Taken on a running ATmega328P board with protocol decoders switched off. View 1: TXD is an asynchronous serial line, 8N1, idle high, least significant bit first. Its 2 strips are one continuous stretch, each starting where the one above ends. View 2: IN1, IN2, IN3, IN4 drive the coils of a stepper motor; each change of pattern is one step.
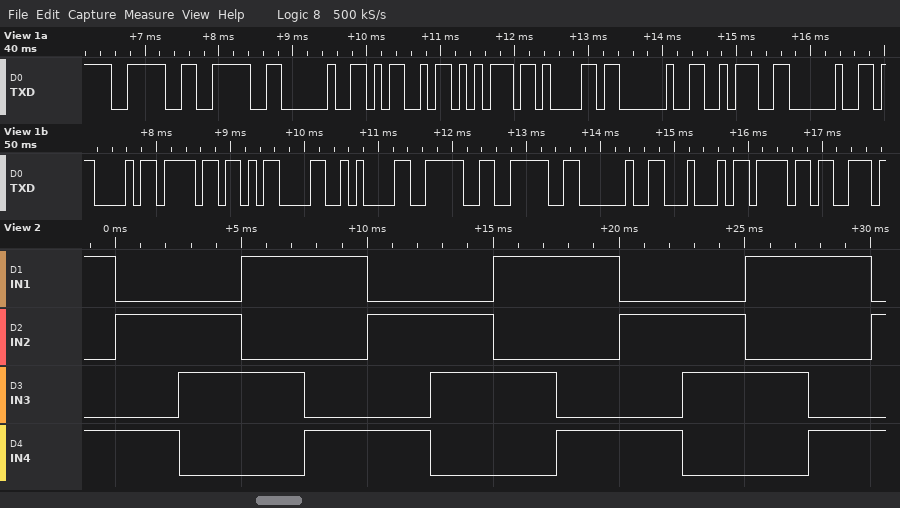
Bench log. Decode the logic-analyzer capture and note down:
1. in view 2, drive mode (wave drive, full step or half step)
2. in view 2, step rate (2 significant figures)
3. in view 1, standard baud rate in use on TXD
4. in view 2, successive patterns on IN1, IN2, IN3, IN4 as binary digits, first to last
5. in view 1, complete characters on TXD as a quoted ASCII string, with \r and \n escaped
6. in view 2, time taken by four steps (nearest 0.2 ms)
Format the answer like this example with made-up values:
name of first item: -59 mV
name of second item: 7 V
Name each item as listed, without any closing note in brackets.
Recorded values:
in view 2, drive mode: full step
in view 2, step rate: 400 steps/s
in view 1, standard baud rate in use on TXD: 9600 baud
in view 2, successive patterns on IN1, IN2, IN3, IN4 as binary digits, first to last: 1001 0101 0110 1010 1001 0101 0110 1010 1001 0101 0110 1010 1001 0101
in view 1, complete characters on TXD as a quoted ASCII string, with \r and \n escaped: ">> Mua : Co\r\n>> Do"
in view 2, time taken by four steps: 10.0 ms
